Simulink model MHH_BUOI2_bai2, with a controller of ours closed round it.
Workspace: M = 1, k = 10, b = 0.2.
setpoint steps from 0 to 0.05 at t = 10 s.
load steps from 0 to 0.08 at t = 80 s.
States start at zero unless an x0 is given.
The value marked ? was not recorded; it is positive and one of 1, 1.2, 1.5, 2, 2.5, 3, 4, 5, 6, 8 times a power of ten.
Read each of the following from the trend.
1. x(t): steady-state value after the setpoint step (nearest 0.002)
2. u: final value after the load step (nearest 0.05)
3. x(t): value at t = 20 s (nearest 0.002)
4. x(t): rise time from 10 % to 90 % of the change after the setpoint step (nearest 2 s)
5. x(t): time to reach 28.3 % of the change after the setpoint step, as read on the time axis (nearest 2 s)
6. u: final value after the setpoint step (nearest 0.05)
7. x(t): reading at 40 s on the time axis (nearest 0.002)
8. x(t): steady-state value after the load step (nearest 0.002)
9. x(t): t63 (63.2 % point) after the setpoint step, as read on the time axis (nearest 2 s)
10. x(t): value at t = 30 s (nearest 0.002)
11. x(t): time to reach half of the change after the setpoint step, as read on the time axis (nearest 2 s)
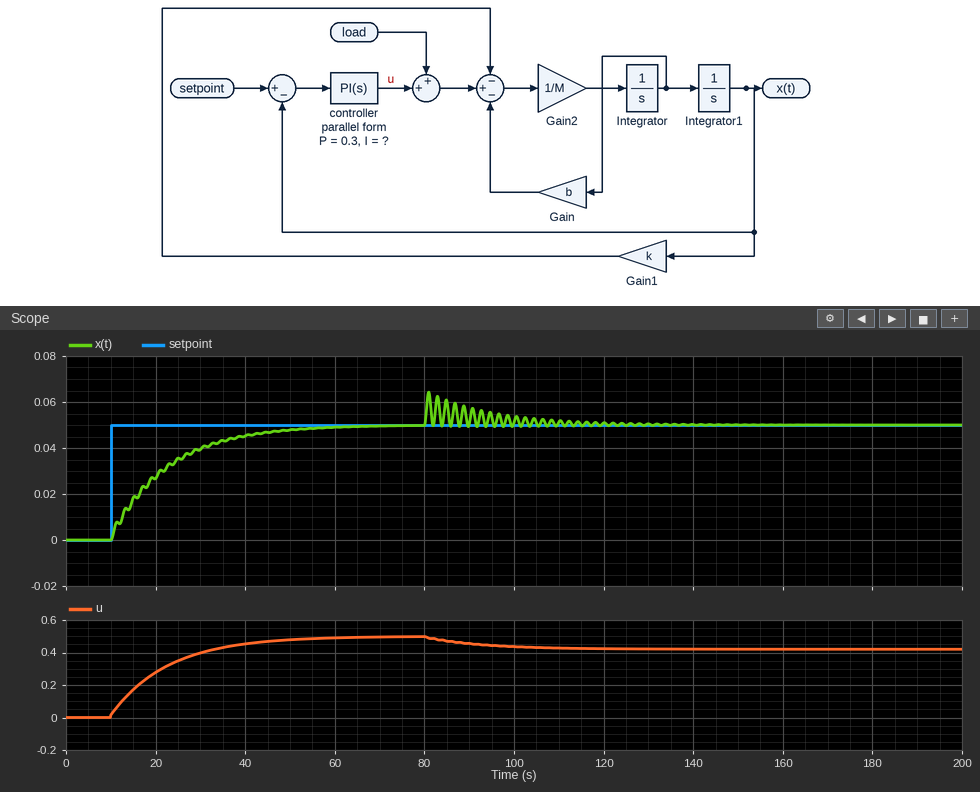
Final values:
0.050
0.40
0.026
28 s
14 s
0.50
0.046
0.050
22 s
0.040
18 s
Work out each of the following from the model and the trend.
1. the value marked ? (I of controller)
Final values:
0.8
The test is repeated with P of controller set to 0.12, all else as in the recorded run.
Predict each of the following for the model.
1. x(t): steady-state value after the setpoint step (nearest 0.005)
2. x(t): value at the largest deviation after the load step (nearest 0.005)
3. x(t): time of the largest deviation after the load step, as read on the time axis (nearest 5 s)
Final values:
0.050
0.065
80 s
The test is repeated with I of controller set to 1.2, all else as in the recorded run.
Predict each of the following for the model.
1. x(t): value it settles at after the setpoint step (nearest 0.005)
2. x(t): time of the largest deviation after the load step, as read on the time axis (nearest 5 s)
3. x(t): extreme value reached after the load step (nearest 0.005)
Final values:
0.050
80 s
0.065
